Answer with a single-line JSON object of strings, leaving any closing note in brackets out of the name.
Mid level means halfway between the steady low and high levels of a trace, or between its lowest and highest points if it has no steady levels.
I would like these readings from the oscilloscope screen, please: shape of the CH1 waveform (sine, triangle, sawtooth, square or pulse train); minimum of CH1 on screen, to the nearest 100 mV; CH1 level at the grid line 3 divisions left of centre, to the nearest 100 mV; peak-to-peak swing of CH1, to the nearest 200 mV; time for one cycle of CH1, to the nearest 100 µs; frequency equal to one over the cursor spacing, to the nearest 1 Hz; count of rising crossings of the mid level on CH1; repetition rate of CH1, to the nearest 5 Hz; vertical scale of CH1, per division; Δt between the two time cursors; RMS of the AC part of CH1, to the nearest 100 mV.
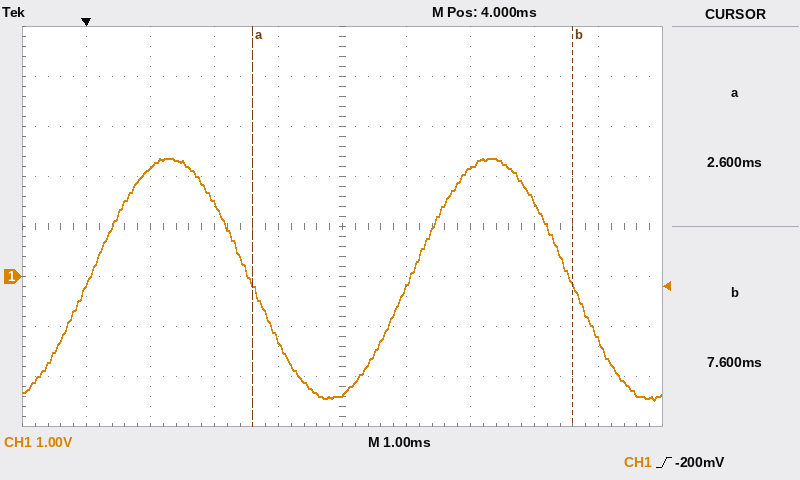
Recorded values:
{"shape of the CH1 waveform": "sine", "minimum of CH1 on screen, to the nearest 100 mV": "-2.5 V", "CH1 level at the grid line 3 divisions left of centre, to the nearest 100 mV": "2.2 V", "peak-to-peak swing of CH1, to the nearest 200 mV": "4.8 V", "time for one cycle of CH1, to the nearest 100 µs": "5.0 ms", "frequency equal to one over the cursor spacing, to the nearest 1 Hz": "200 Hz", "count of rising crossings of the mid level on CH1": "2", "repetition rate of CH1, to the nearest 5 Hz": "200 Hz", "vertical scale of CH1, per division": "1 V", "Δt between the two time cursors": "5.0 ms", "RMS of the AC part of CH1, to the nearest 100 mV": "1.7 V"}
